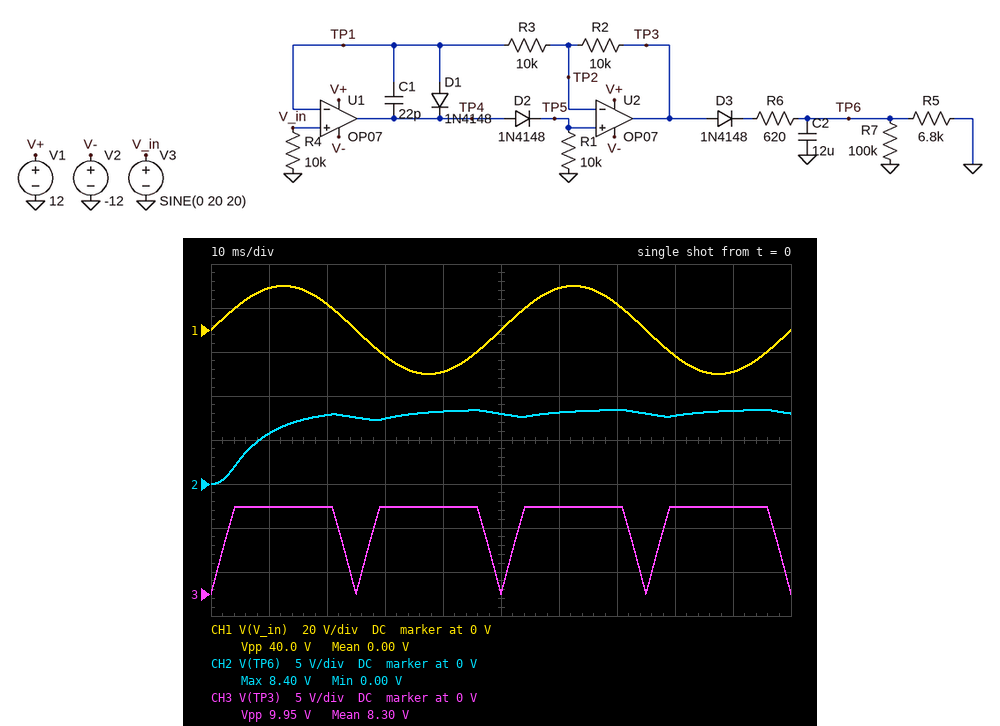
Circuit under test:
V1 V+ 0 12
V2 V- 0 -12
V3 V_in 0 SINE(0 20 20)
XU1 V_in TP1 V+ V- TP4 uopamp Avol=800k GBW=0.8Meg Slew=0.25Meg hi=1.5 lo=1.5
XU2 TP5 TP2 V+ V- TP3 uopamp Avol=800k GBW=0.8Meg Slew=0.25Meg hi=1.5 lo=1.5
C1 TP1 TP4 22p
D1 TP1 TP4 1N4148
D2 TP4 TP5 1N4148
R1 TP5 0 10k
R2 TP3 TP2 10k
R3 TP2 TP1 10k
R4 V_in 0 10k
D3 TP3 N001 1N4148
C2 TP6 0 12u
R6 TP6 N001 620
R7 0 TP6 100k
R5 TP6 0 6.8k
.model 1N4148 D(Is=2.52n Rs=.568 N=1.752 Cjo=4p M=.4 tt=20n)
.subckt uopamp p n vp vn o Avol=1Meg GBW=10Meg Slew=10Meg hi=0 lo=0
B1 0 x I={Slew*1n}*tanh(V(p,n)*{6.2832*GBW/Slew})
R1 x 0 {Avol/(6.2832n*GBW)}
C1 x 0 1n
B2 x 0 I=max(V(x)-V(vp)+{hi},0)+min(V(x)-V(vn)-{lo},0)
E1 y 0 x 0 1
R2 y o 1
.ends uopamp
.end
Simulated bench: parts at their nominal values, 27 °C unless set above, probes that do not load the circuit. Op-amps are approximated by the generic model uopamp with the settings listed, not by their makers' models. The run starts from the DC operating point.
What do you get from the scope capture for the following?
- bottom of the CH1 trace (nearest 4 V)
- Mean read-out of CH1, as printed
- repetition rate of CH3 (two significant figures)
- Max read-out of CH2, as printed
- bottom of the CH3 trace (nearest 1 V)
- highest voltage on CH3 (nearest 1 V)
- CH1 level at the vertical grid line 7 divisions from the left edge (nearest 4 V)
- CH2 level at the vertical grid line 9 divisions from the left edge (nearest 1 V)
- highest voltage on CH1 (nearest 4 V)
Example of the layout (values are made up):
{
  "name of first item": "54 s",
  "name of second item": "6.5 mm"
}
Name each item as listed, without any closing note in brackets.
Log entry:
{
  "bottom of the CH1 trace": "-20 V",
  "Mean read-out of CH1, as printed": "0.00 V",
  "repetition rate of CH3": "40 Hz",
  "Max read-out of CH2, as printed": "8.40 V",
  "bottom of the CH3 trace": "0 V",
  "highest voltage on CH3": "10 V",
  "CH1 level at the vertical grid line 7 divisions from the left edge": "12 V",
  "CH2 level at the vertical grid line 9 divisions from the left edge": "8 V",
  "highest voltage on CH1": "20 V"
}
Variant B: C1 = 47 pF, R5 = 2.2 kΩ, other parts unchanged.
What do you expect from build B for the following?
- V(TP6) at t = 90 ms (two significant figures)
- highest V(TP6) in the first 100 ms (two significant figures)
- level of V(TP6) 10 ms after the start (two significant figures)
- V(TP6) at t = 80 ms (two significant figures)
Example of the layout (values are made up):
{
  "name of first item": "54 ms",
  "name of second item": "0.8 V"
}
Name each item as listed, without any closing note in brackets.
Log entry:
{
  "V(TP6) at t = 90 ms": "7.0 V",
  "highest V(TP6) in the first 100 ms": "7.1 V",
  "level of V(TP6) 10 ms after the start": "5.3 V",
  "V(TP6) at t = 80 ms": "5.9 V"
}
